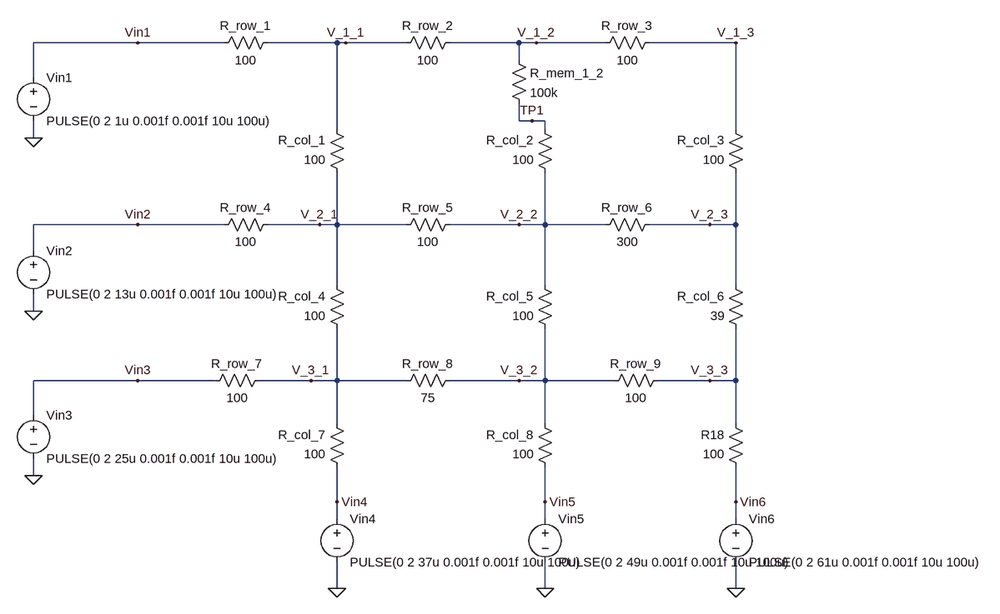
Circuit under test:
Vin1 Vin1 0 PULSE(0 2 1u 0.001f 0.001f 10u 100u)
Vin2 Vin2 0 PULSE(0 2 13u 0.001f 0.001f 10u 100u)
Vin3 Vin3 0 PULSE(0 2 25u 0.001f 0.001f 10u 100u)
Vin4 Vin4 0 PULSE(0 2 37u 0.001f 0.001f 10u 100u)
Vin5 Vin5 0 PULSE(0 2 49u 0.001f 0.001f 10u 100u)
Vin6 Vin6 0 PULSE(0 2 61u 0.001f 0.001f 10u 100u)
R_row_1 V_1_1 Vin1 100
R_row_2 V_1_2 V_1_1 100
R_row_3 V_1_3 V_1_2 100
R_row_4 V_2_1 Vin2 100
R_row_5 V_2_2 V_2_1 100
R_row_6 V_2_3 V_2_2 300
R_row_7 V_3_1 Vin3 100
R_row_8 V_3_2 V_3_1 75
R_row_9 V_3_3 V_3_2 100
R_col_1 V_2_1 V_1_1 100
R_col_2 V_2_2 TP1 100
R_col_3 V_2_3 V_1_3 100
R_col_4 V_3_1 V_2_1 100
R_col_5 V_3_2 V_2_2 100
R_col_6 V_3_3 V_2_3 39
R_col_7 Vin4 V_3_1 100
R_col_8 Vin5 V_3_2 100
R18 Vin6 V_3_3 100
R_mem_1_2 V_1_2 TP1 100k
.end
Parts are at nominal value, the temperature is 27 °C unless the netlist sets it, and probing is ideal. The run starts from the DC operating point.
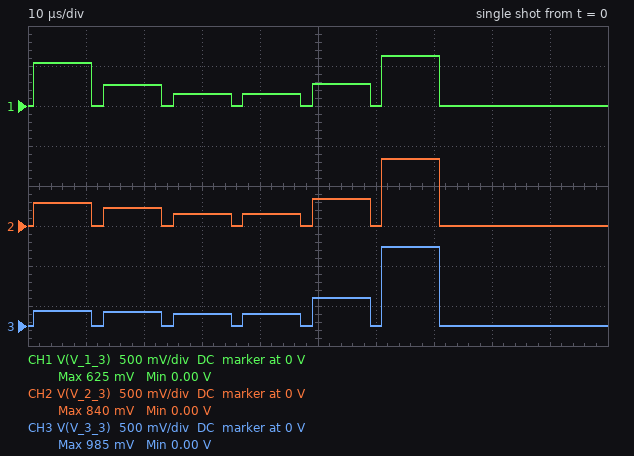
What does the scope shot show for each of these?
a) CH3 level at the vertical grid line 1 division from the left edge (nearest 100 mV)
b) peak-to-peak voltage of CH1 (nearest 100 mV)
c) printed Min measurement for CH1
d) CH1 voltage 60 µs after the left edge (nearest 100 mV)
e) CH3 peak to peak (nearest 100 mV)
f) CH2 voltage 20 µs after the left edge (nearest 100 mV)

200 mV
600 mV
0.00 V
0 V
1.0 V
200 mV
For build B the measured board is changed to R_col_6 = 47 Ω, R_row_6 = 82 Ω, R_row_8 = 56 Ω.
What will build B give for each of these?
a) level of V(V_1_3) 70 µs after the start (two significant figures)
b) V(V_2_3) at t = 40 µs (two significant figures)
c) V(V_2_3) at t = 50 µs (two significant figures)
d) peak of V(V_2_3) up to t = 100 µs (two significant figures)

530 mV
190 mV
350 mV
700 mV
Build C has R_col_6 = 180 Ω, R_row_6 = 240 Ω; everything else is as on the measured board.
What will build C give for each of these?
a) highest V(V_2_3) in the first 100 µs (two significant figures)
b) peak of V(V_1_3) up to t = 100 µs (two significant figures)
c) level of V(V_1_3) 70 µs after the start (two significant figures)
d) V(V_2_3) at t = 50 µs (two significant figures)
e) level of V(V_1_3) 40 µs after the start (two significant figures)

580 mV
650 mV
440 mV
330 mV
160 mV
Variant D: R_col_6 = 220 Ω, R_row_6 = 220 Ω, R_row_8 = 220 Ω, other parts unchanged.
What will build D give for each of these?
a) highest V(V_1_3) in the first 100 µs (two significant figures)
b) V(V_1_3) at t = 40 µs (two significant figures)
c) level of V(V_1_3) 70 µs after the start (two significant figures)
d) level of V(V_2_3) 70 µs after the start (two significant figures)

660 mV
140 mV
420 mV
560 mV
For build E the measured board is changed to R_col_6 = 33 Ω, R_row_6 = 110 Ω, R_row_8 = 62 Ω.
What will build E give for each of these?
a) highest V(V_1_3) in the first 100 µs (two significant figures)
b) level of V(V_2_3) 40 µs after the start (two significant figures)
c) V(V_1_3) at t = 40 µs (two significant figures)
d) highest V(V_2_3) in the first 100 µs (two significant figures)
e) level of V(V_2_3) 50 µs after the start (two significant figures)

570 mV
180 mV
160 mV
760 mV
350 mV
